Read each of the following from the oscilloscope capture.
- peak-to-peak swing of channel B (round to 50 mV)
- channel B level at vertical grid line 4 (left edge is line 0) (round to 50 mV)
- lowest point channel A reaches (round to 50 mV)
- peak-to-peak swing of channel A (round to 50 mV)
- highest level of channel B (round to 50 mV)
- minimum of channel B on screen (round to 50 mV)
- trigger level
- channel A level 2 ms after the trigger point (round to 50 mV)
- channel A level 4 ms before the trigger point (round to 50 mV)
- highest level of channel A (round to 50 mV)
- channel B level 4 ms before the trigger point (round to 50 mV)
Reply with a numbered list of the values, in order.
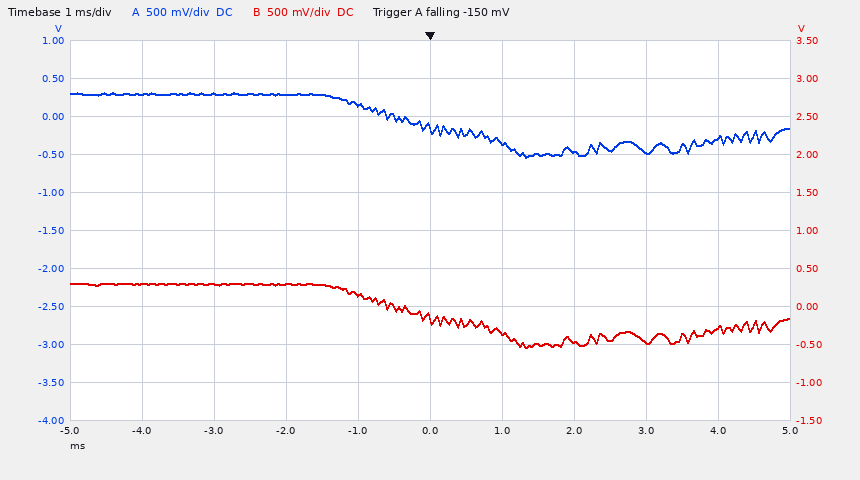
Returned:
1. 850 mV
2. 150 mV
3. -550 mV
4. 850 mV
5. 300 mV
6. -550 mV
7. -150 mV
8. -450 mV
9. 300 mV
10. 300 mV
11. 300 mV
